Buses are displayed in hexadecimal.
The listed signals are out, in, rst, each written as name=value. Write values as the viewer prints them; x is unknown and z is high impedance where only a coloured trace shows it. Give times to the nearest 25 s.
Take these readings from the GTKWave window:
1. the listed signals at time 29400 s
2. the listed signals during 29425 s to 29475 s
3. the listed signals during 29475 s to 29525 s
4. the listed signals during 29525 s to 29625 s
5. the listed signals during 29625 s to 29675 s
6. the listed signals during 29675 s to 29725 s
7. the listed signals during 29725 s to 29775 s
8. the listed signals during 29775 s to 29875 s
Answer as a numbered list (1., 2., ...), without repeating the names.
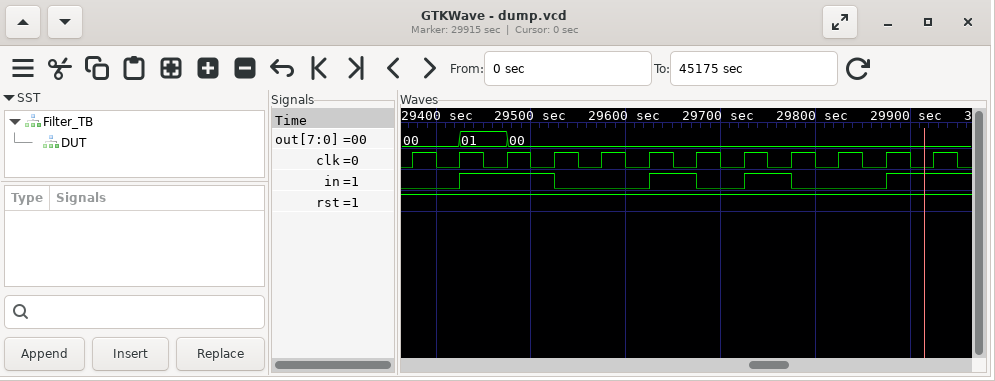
1. out=00, in=0, rst=1
2. out=01, in=1, rst=1
3. out=00, in=1, rst=1
4. out=00, in=0, rst=1
5. out=00, in=1, rst=1
6. out=00, in=0, rst=1
7. out=00, in=1, rst=1
8. out=00, in=0, rst=1
